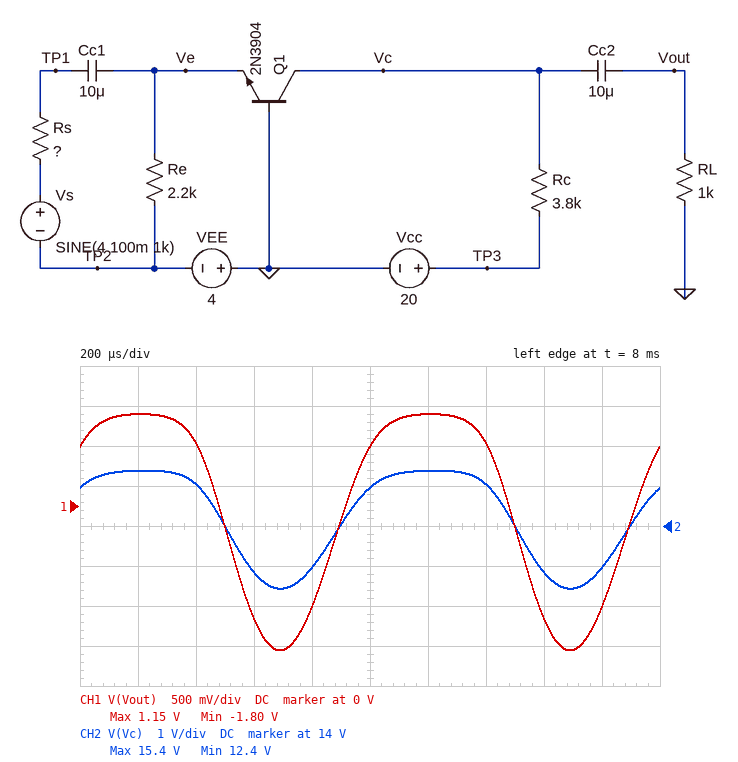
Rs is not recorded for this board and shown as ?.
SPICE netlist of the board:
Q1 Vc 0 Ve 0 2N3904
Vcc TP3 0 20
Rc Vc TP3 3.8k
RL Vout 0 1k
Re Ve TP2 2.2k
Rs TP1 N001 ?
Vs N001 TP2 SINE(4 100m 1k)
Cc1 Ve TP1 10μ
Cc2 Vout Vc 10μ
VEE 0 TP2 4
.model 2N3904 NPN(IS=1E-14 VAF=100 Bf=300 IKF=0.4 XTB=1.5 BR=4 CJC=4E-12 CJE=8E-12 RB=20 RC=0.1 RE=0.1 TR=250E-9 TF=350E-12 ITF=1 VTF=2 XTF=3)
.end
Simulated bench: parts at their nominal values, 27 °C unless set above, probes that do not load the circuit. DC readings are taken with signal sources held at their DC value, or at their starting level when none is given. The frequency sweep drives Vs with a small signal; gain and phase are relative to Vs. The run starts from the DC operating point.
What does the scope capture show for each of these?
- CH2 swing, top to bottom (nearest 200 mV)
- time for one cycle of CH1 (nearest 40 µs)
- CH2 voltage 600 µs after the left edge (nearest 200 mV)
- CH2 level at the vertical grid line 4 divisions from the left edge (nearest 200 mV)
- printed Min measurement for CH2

3.0 V
1.00 ms
12.8 V
13.0 V
12.4 V
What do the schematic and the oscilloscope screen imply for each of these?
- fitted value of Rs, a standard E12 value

22 Ω
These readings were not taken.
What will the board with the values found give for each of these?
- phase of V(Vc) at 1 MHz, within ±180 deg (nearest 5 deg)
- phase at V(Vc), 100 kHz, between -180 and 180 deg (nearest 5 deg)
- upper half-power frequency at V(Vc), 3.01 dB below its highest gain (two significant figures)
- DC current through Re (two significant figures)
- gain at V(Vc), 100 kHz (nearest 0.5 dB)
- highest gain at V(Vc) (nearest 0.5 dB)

0 deg
0 deg
75 MHz
1.5 mA
26.0 dB
26.0 dB
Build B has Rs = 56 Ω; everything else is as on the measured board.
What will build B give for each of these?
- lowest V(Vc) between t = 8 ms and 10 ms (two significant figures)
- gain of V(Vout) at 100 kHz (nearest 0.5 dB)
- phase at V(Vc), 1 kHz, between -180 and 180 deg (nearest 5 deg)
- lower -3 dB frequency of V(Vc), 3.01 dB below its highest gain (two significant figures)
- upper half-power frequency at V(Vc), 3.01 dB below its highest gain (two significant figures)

13 V
20.5 dB
10 deg
220 Hz
88 MHz
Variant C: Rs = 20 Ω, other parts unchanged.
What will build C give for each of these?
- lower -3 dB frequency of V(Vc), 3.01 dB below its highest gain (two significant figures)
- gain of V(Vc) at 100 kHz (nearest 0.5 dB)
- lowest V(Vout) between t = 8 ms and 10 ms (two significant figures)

430 Hz
26.5 dB
-1.9 V
